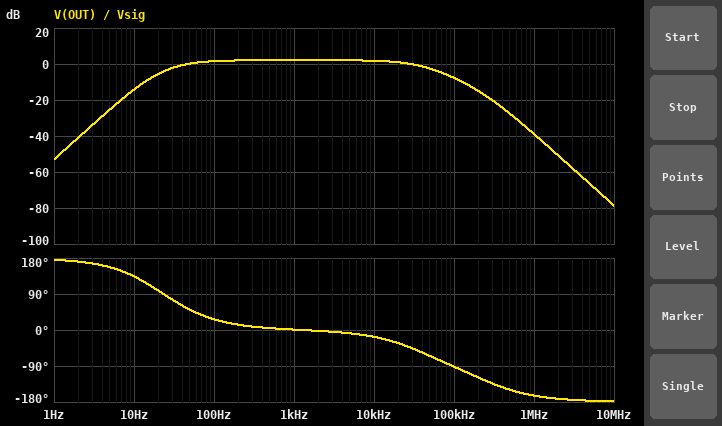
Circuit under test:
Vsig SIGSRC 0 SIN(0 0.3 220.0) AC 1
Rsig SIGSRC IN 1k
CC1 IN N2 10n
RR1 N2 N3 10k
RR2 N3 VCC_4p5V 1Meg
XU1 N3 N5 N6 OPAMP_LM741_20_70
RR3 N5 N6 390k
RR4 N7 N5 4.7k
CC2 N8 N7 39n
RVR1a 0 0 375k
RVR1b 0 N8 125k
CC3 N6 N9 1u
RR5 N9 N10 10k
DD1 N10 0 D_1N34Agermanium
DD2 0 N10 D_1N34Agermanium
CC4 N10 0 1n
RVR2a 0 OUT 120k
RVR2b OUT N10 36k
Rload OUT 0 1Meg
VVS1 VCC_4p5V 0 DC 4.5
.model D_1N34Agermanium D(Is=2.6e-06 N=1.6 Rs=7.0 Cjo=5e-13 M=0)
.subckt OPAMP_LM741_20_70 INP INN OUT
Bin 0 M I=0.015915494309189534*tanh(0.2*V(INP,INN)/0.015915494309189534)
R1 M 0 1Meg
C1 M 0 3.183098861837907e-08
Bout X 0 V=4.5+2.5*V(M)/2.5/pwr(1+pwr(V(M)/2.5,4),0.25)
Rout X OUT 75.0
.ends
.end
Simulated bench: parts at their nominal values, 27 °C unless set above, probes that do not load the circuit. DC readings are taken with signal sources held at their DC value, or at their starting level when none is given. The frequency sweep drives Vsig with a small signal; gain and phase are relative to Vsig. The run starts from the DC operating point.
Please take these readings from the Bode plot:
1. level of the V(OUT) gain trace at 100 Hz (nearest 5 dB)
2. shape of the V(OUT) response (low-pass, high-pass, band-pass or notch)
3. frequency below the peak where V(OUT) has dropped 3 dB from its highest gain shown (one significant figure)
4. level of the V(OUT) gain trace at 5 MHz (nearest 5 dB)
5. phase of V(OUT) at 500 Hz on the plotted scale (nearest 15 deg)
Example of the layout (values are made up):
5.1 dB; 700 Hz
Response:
0 dB; band-pass; 40 Hz; -65 dB; 0 deg
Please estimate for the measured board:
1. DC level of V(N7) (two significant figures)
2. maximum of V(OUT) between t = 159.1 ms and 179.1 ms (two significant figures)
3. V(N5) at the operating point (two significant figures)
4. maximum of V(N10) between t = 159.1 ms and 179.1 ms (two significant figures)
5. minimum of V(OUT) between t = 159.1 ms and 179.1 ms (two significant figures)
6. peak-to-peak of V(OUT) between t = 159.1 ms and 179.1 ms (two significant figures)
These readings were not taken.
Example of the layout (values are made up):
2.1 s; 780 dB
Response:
4.5 V; 110 mV; 4.5 V; 150 mV; -110 mV; 230 mV
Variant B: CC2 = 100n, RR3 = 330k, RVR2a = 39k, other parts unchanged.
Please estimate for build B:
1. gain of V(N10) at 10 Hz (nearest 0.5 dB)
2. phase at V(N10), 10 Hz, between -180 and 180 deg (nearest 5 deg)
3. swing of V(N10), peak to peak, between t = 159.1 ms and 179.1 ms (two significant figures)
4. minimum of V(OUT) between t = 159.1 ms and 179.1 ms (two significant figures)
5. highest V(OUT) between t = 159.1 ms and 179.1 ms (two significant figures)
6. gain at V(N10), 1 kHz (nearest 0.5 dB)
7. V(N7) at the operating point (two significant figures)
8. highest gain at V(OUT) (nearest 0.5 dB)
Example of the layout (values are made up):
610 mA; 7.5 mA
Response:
-8.5 dB; 130 deg; 290 mV; -75 mV; 75 mV; 3.5 dB; 4.5 V; -2.5 dB
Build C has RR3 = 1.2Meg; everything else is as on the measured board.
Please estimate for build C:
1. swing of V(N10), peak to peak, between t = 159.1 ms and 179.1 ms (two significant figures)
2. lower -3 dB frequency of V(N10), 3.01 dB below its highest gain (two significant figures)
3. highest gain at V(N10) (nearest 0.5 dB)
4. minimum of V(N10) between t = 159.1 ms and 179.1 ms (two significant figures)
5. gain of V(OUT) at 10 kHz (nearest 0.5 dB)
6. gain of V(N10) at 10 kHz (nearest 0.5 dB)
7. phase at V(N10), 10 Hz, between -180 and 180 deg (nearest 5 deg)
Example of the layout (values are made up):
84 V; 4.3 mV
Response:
380 mV; 39 Hz; 13.0 dB; -190 mV; 10.0 dB; 12.5 dB; 155 deg
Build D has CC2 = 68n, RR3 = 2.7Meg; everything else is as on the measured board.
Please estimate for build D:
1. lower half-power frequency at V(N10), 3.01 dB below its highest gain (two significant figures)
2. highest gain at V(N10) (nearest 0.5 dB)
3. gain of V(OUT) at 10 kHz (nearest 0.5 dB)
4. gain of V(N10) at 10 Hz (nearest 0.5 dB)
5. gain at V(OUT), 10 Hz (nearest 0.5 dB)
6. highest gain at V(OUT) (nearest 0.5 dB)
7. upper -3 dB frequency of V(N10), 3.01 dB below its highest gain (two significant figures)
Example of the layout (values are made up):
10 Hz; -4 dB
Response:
29 Hz; 19.5 dB; 16.5 dB; 5.0 dB; 2.5 dB; 17.0 dB; 26 kHz
